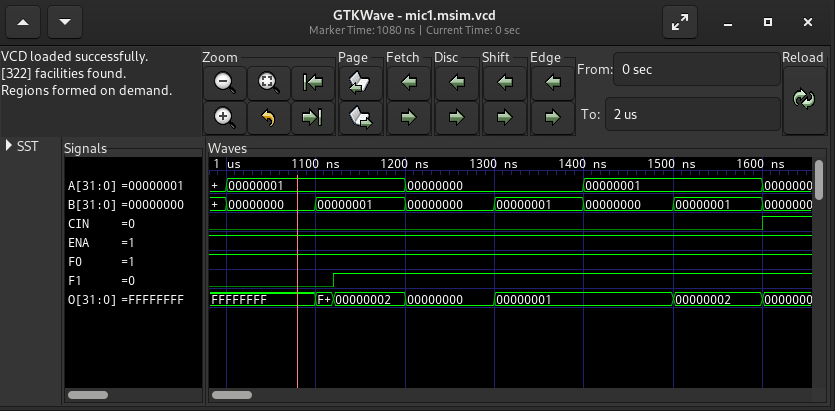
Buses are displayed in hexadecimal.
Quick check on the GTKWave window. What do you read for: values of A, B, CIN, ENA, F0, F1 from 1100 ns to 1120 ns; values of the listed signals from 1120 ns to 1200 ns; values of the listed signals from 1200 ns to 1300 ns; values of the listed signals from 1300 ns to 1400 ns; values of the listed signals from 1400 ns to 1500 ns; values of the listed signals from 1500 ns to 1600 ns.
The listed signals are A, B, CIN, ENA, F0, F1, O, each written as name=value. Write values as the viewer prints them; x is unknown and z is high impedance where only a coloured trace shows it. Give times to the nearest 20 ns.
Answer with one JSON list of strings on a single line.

["A=00000001, B=00000001, CIN=0, ENA=1, F0=1, F1=0", "A=00000001, B=00000001, CIN=0, ENA=1, F0=1, F1=1, O=00000002", "A=00000000, B=00000000, CIN=0, ENA=1, F0=1, F1=1, O=00000000", "A=00000000, B=00000001, CIN=0, ENA=1, F0=1, F1=1, O=00000001", "A=00000001, B=00000000, CIN=0, ENA=1, F0=1, F1=1, O=00000001", "A=00000001, B=00000001, CIN=0, ENA=1, F0=1, F1=1, O=00000002"]
